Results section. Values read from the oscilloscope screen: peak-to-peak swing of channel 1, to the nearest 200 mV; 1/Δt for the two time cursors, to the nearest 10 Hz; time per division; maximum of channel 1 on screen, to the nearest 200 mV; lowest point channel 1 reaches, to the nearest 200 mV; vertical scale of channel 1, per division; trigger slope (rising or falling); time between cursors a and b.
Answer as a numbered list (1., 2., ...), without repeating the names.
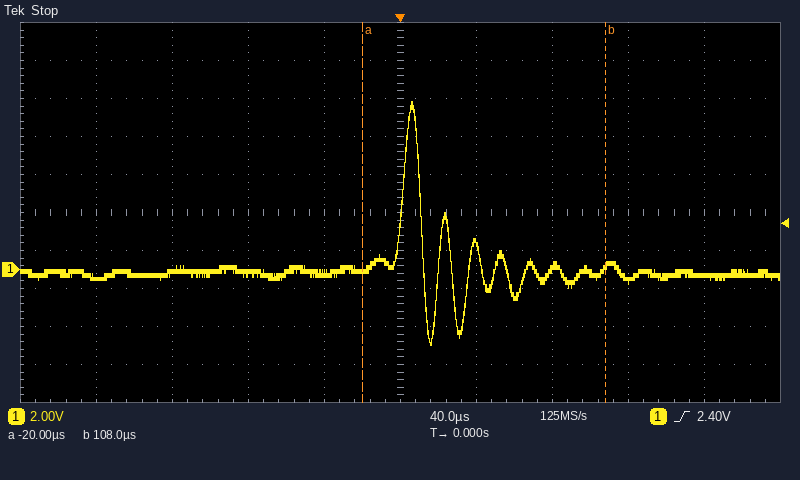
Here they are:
1. 12.8 V
2. 7.81 kHz
3. 40 µs
4. 8.8 V
5. -4.0 V
6. 2 V
7. rising
8. 128 µs
